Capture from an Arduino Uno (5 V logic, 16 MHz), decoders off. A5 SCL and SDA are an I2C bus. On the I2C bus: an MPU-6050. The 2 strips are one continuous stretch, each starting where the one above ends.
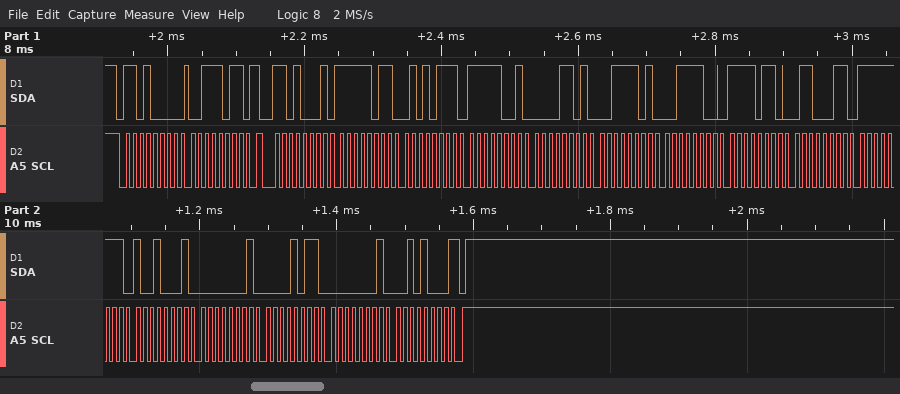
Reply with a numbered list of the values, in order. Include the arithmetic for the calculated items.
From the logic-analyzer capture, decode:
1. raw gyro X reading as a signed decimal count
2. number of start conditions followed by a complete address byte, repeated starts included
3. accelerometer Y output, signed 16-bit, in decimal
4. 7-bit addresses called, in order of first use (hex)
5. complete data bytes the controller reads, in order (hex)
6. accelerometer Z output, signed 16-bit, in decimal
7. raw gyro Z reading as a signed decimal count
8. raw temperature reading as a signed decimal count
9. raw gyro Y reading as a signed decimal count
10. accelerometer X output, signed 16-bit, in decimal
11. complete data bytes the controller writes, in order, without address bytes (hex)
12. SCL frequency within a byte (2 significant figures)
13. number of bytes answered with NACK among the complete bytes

1. 0xFF91 = -111
2. 2
3. 0xF90D = -1779
4. 0x68
5. FB 57 F9 0D 3D 3C F6 63 FF 91 01 0B 01 28
6. 0x3D3C = 15676
7. 0x0128 = 296
8. 0xF663 = -2461
9. 0x010B = 267
10. 0xFB57 = -1193
11. 3B
12. 100 kHz
13. 1
